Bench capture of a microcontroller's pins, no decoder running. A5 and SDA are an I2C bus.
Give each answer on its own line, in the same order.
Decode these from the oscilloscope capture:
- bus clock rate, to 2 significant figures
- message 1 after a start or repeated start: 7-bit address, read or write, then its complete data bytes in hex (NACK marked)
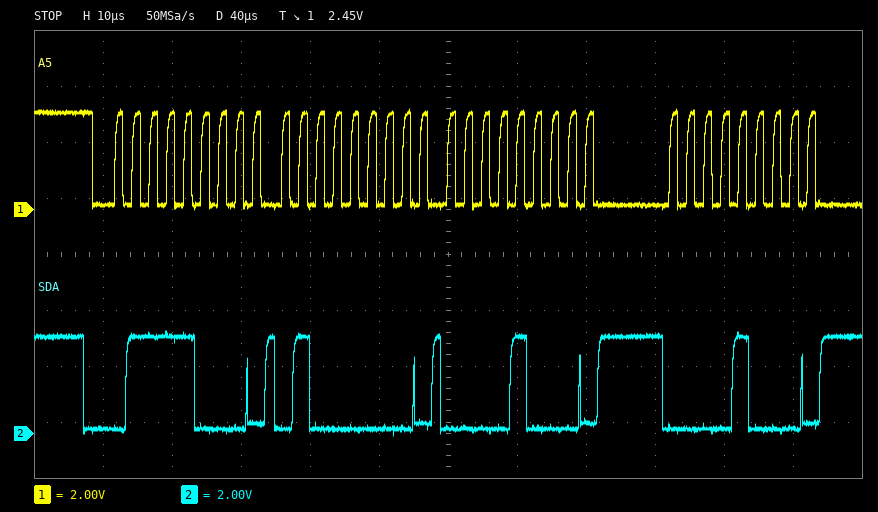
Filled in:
400 kHz
0x3C write: 40 08 08
